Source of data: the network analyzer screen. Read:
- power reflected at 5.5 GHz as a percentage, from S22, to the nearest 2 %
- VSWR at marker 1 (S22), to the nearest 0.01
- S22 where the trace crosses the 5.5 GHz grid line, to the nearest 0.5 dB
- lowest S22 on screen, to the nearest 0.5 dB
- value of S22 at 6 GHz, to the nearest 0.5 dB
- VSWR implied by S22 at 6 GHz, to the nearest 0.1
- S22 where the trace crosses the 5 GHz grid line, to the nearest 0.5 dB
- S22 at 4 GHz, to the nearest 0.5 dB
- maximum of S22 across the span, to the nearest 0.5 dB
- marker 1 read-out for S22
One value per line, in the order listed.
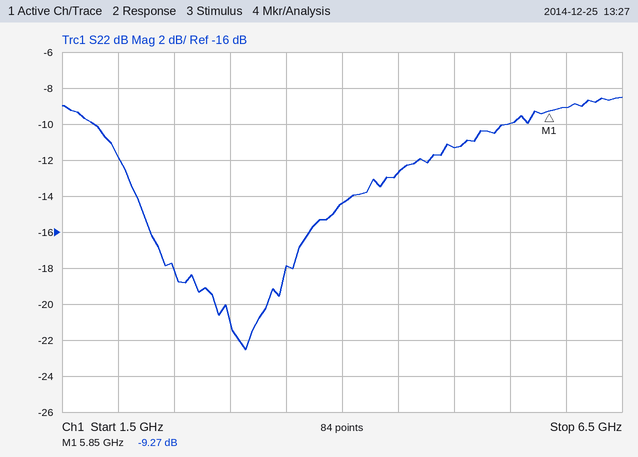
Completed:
10 %
2.05
-10.0 dB
-22.5 dB
-9.0 dB
2.1
-11.5 dB
-14.5 dB
-8.5 dB
-9.27 dB
